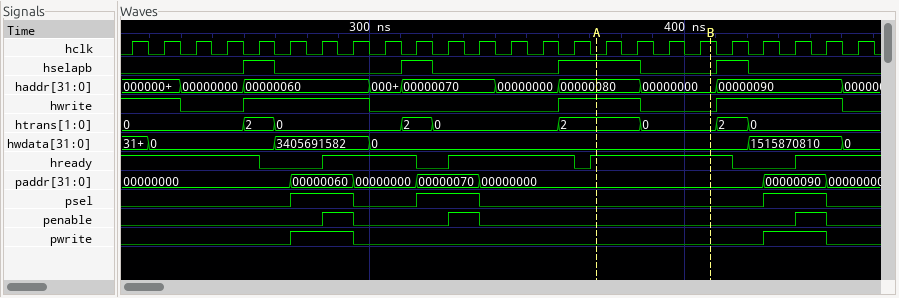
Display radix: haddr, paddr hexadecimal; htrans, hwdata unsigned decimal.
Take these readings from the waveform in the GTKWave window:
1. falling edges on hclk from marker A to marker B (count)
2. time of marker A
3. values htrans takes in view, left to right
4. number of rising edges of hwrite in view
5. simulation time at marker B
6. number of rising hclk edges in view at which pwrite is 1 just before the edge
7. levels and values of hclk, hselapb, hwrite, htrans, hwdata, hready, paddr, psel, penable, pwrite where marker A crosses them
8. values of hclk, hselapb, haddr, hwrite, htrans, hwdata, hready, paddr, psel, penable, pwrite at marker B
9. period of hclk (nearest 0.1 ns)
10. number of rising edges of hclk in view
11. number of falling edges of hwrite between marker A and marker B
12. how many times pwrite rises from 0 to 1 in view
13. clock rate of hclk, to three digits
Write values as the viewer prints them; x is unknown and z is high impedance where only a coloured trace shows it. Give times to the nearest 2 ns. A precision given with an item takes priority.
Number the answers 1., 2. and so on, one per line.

1. 3
2. 372 ns
3. 0, 2, 0, 2, 0, 2, 0, 2, 0
4. 3
5. 408 ns
6. 4
7. hclk=0, hselapb=1, hwrite=1, htrans=2, hwdata=0, hready=1, paddr=00000000, psel=0, penable=0, pwrite=0
8. hclk=1, hselapb=0, haddr=00000000, hwrite=0, htrans=0, hwdata=0, hready=1, paddr=00000000, psel=0, penable=0, pwrite=0
9. 10 ns
10. 24
11. 1
12. 2
13. 100 MHz
